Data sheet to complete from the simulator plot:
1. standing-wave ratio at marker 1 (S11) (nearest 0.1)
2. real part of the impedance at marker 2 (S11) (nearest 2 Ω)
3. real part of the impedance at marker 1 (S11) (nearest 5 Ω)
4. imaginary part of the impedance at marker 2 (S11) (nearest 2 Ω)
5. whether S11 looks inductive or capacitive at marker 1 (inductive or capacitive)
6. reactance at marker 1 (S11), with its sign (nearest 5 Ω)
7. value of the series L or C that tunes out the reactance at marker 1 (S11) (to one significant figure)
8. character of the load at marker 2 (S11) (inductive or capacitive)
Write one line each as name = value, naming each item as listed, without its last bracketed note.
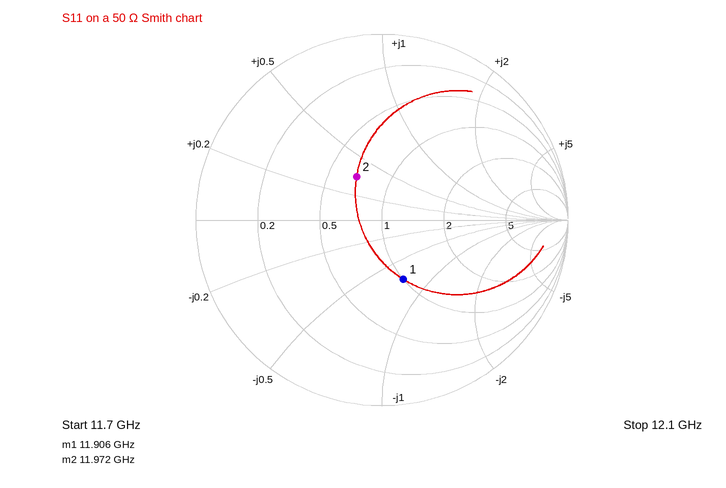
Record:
standing-wave ratio at marker 1 (S11) = 2.0
real part of the impedance at marker 2 (S11) = 34 Ω
real part of the impedance at marker 1 (S11) = 50 Ω
imaginary part of the impedance at marker 2 (S11) = +18 Ω
whether S11 looks inductive or capacitive at marker 1 = capacitive
reactance at marker 1 (S11), with its sign = -35 Ω
value of the series L or C that tunes out the reactance at marker 1 (S11) = 500 pH
character of the load at marker 2 (S11) = inductive
